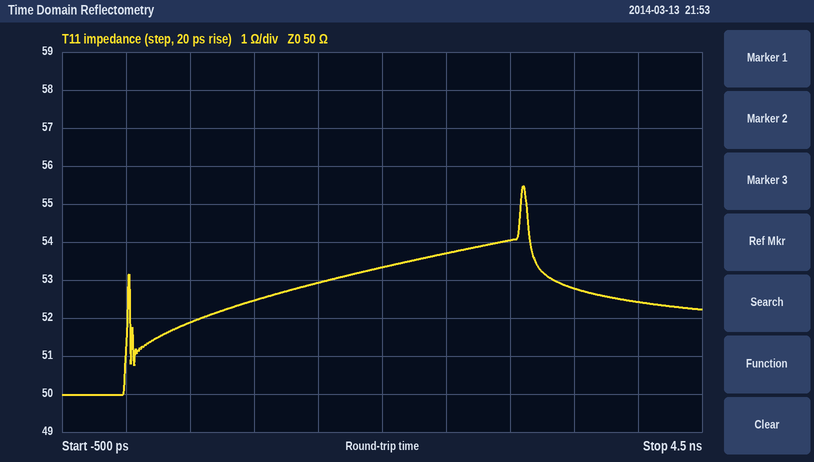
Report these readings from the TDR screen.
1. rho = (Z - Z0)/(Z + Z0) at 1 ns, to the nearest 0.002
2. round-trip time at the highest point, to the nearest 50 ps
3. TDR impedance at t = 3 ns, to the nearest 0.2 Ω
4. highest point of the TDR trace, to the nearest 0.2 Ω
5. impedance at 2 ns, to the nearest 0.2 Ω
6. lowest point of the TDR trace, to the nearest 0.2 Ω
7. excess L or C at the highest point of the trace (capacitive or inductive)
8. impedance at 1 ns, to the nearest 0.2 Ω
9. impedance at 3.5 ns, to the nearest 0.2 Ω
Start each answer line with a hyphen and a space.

- +0.024
- 3.10 ns
- 54.0 Ω
- 55.4 Ω
- 53.4 Ω
- 50.0 Ω
- inductive
- 52.4 Ω
- 52.8 Ω
